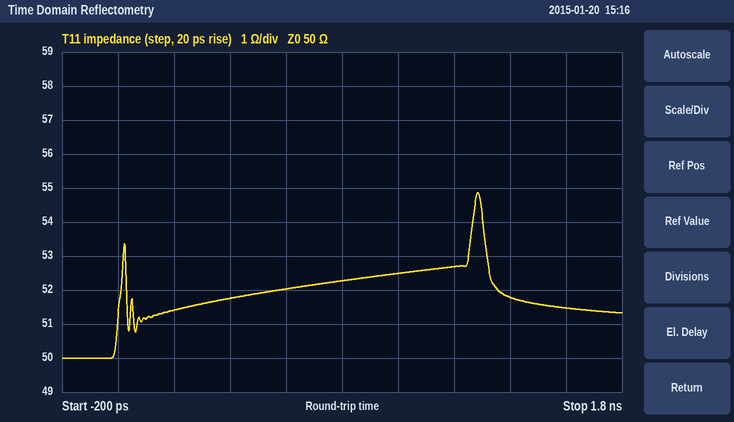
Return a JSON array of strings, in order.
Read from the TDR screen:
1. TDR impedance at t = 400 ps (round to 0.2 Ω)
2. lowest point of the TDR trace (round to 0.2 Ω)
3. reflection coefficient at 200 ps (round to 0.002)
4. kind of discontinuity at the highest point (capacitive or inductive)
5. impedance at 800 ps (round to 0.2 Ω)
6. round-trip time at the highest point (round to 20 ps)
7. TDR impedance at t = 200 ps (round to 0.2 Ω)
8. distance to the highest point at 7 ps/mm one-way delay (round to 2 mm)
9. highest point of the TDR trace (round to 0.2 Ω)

["51.8 Ω", "50.0 Ω", "+0.014", "inductive", "52.2 Ω", "1.28 ns", "51.4 Ω", "92 mm", "54.8 Ω"]
